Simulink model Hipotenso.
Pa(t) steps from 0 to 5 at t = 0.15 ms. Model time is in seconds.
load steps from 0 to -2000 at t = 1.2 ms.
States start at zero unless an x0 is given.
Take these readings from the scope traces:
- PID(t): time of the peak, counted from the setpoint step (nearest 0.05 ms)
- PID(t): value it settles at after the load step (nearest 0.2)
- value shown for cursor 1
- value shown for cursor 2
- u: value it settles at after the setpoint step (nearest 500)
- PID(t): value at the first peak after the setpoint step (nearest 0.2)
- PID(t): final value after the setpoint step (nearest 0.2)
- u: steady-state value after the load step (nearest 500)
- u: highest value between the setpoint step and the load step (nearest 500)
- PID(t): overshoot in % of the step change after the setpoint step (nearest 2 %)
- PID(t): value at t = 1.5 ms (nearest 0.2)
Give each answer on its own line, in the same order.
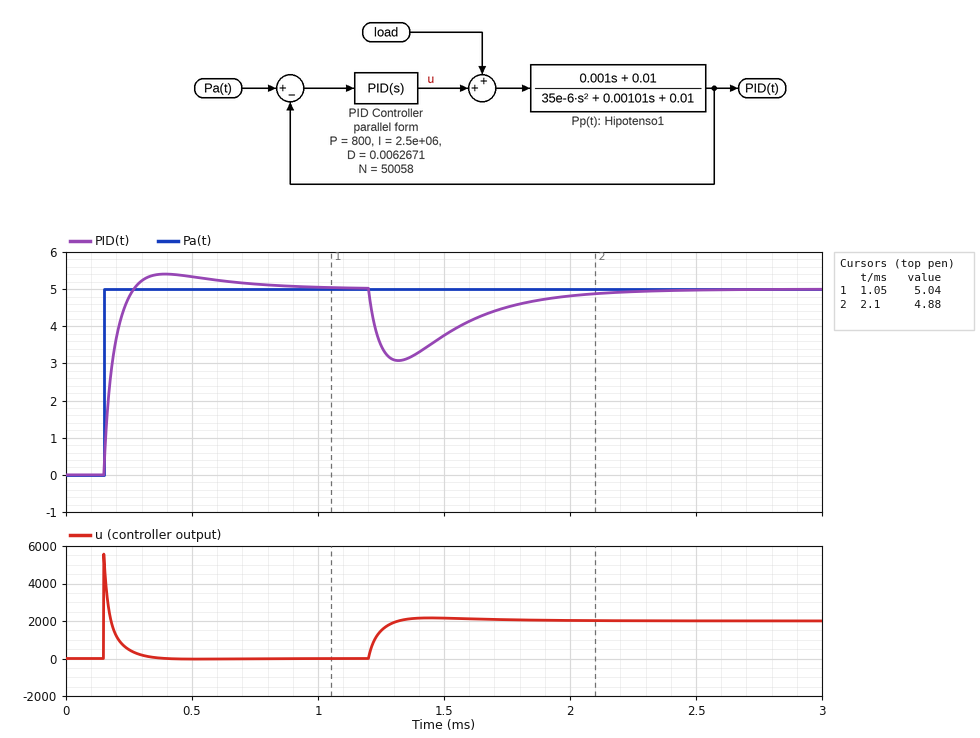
0.25 ms
5.0
5.04
4.88
0
5.4
5.0
2000
5500
8 %
3.8
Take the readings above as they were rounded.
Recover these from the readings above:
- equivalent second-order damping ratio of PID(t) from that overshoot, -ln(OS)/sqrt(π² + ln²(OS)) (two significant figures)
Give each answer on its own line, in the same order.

0.63
